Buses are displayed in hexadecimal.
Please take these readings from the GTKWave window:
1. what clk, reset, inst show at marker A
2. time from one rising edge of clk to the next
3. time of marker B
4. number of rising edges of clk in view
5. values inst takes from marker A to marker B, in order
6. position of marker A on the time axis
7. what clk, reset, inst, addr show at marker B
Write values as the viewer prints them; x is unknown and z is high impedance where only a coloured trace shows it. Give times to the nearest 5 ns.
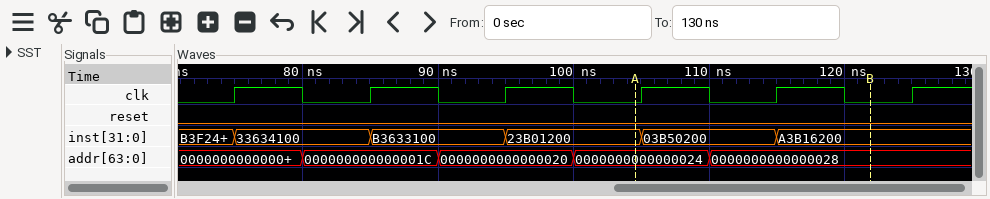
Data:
clk=0, reset=0, inst=23B01200
10 ns
120 ns
6
23B01200, 03B50200, A3B16200
105 ns
clk=0, reset=0, inst=A3B16200, addr=0000000000000028
